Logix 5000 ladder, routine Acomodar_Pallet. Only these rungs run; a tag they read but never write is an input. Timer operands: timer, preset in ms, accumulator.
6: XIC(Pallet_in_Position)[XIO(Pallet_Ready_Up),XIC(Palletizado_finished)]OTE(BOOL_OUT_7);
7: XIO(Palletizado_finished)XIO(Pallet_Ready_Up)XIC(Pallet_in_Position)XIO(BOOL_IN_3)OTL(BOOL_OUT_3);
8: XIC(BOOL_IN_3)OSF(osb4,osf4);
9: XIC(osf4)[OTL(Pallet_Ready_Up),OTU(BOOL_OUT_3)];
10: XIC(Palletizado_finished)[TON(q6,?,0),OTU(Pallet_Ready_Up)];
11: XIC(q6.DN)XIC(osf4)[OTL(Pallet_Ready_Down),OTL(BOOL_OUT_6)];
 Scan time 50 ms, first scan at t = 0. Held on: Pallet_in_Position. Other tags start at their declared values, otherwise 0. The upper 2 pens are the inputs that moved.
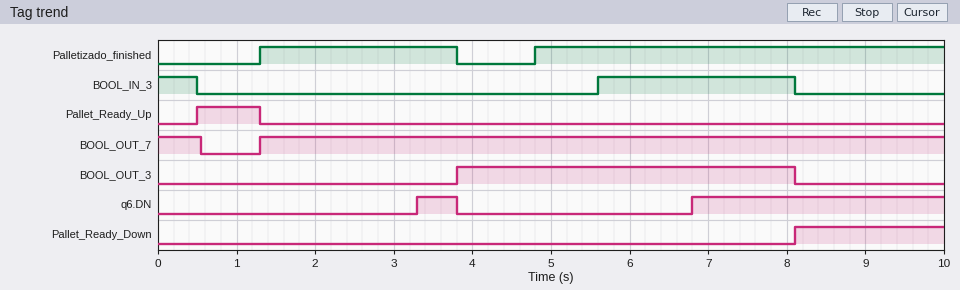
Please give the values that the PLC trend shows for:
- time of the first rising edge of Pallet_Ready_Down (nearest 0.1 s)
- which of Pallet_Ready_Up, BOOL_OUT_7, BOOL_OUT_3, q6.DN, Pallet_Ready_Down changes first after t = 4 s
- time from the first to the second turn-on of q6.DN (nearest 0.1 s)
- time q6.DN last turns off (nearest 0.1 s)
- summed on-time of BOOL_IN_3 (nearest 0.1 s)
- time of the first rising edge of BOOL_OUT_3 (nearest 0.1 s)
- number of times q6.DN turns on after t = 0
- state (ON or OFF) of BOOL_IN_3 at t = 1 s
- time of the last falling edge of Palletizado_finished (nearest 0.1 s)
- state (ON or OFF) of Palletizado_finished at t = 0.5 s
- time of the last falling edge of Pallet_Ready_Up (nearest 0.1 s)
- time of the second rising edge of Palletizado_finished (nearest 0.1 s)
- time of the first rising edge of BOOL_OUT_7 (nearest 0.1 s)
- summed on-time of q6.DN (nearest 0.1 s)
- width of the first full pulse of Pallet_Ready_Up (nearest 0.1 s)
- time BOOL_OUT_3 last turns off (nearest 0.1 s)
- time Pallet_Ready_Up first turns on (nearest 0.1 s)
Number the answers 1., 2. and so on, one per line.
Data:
1. 8.1 s
2. q6.DN
3. 3.5 s
4. 3.8 s
5. 3.0 s
6. 3.8 s
7. 2
8. OFF
9. 3.8 s
10. OFF
11. 1.3 s
12. 4.8 s
13. 1.3 s
14. 3.7 s
15. 0.8 s
16. 8.1 s
17. 0.5 s
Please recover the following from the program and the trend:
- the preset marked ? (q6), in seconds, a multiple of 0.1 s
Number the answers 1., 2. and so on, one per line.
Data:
1. 2.0 s
